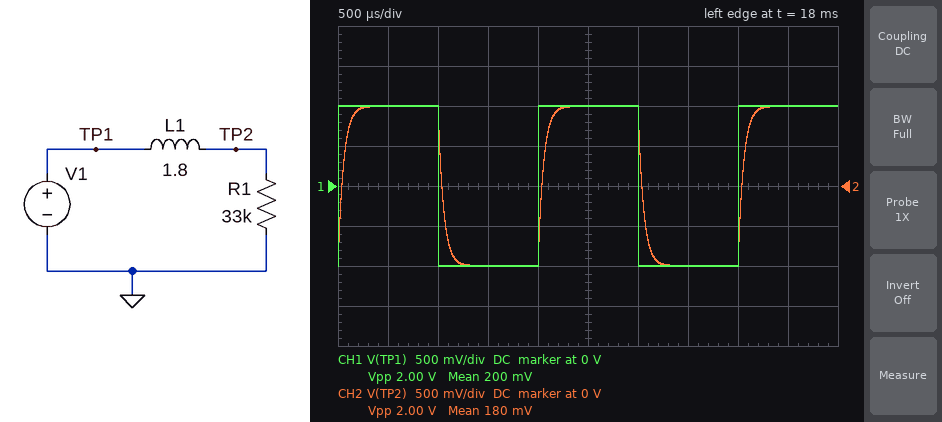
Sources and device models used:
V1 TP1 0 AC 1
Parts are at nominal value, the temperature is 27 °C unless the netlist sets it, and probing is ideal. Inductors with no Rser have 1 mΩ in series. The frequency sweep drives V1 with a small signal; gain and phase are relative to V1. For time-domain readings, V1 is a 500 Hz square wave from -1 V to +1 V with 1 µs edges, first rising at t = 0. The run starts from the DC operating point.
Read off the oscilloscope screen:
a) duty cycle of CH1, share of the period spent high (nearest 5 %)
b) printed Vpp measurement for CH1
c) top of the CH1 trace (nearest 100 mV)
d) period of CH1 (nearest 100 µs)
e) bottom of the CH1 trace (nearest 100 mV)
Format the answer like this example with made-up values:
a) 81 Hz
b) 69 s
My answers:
a) 50 %
b) 2.00 V
c) 1.0 V
d) 2.0 ms
e) -1.0 V
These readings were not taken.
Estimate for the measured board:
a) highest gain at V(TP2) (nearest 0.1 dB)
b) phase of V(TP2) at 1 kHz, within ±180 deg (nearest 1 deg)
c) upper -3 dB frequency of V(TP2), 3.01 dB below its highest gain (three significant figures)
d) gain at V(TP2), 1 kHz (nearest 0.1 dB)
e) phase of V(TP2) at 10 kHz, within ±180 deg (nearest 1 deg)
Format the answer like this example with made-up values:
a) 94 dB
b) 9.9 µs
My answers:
a) 0 dB
b) -19 deg
c) 2.92 kHz
d) -0.5 dB
e) -74 deg
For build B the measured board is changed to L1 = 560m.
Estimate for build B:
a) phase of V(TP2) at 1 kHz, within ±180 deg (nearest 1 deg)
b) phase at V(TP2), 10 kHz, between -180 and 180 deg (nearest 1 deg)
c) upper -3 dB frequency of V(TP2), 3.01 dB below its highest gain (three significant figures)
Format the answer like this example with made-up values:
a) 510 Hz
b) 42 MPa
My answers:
a) -6 deg
b) -47 deg
c) 9.38 kHz
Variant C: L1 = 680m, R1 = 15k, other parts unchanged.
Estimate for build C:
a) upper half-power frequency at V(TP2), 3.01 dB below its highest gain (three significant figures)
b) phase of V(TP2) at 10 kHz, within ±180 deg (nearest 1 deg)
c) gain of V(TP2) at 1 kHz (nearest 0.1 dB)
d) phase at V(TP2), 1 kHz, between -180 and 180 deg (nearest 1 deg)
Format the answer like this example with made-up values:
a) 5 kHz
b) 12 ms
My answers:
a) 3.51 kHz
b) -71 deg
c) -0.3 dB
d) -16 deg
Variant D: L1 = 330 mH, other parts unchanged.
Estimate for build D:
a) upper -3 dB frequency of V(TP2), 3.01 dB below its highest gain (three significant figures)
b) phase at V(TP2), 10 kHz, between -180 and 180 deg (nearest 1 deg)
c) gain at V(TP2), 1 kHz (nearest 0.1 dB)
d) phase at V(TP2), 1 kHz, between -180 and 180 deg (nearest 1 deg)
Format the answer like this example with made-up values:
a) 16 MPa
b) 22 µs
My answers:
a) 15.9 kHz
b) -32 deg
c) 0 dB
d) -4 deg
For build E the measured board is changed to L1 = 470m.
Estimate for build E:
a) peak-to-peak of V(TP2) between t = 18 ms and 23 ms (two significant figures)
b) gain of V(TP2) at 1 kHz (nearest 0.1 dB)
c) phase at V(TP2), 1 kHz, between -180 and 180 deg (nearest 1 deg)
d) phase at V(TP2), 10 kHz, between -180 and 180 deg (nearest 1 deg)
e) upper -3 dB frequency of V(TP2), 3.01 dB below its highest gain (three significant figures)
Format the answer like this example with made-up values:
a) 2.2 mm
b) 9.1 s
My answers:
a) 2.0 V
b) 0 dB
c) -5 deg
d) -42 deg
e) 11.2 kHz
